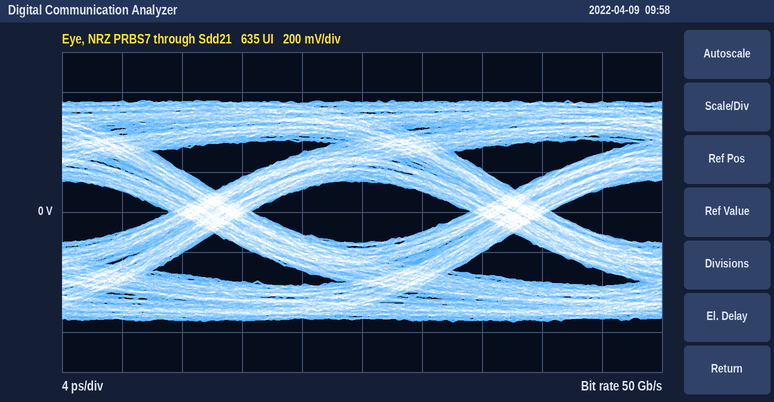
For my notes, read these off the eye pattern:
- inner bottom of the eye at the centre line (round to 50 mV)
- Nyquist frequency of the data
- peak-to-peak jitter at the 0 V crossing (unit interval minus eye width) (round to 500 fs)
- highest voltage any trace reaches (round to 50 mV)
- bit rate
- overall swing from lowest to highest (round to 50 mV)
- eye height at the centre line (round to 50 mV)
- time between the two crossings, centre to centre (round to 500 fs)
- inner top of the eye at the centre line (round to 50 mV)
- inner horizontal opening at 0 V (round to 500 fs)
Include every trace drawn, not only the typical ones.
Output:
-150 mV
25 GHz
5.5 ps
550 mV
50 Gb/s
1.10 V
300 mV
20.0 ps
150 mV
14.5 ps
